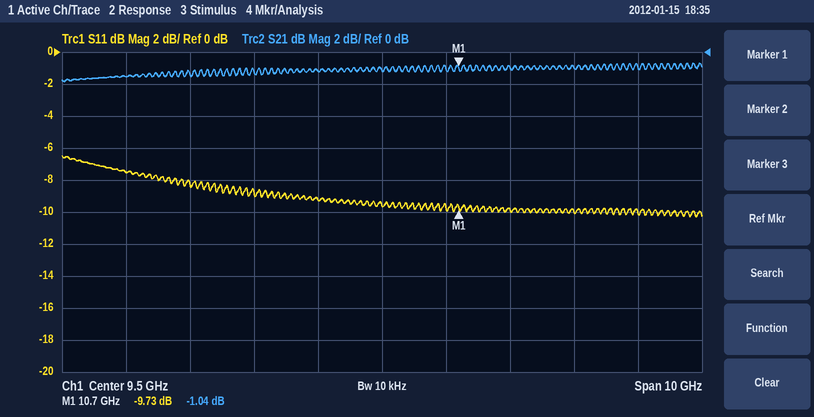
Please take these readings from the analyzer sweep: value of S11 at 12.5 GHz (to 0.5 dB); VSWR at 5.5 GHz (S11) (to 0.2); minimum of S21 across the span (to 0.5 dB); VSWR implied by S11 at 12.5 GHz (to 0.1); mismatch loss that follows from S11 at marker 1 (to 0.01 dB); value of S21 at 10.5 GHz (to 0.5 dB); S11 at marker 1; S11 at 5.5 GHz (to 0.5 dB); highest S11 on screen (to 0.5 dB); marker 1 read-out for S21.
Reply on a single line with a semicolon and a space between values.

-10.0 dB; 2.4; -2.0 dB; 1.9; 0.49 dB; -1.0 dB; -9.73 dB; -7.5 dB; -6.5 dB; -1.04 dB
